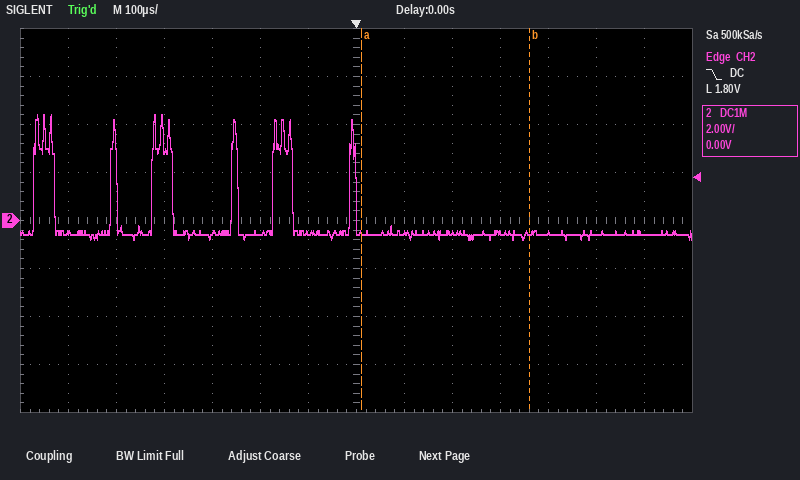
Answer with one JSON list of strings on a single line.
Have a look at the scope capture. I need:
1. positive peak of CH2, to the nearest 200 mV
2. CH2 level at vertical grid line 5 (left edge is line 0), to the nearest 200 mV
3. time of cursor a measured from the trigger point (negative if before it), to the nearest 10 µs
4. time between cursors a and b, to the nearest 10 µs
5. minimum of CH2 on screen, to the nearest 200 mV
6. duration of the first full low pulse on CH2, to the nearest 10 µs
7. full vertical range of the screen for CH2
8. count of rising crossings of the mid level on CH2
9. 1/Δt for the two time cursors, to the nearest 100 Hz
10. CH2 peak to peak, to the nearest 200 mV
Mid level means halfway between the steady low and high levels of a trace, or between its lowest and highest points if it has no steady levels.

["4.4 V", "-600 mV", "+10 µs", "350 µs", "-800 mV", "120 µs", "16 V", "6", "2.9 kHz", "5.2 V"]
